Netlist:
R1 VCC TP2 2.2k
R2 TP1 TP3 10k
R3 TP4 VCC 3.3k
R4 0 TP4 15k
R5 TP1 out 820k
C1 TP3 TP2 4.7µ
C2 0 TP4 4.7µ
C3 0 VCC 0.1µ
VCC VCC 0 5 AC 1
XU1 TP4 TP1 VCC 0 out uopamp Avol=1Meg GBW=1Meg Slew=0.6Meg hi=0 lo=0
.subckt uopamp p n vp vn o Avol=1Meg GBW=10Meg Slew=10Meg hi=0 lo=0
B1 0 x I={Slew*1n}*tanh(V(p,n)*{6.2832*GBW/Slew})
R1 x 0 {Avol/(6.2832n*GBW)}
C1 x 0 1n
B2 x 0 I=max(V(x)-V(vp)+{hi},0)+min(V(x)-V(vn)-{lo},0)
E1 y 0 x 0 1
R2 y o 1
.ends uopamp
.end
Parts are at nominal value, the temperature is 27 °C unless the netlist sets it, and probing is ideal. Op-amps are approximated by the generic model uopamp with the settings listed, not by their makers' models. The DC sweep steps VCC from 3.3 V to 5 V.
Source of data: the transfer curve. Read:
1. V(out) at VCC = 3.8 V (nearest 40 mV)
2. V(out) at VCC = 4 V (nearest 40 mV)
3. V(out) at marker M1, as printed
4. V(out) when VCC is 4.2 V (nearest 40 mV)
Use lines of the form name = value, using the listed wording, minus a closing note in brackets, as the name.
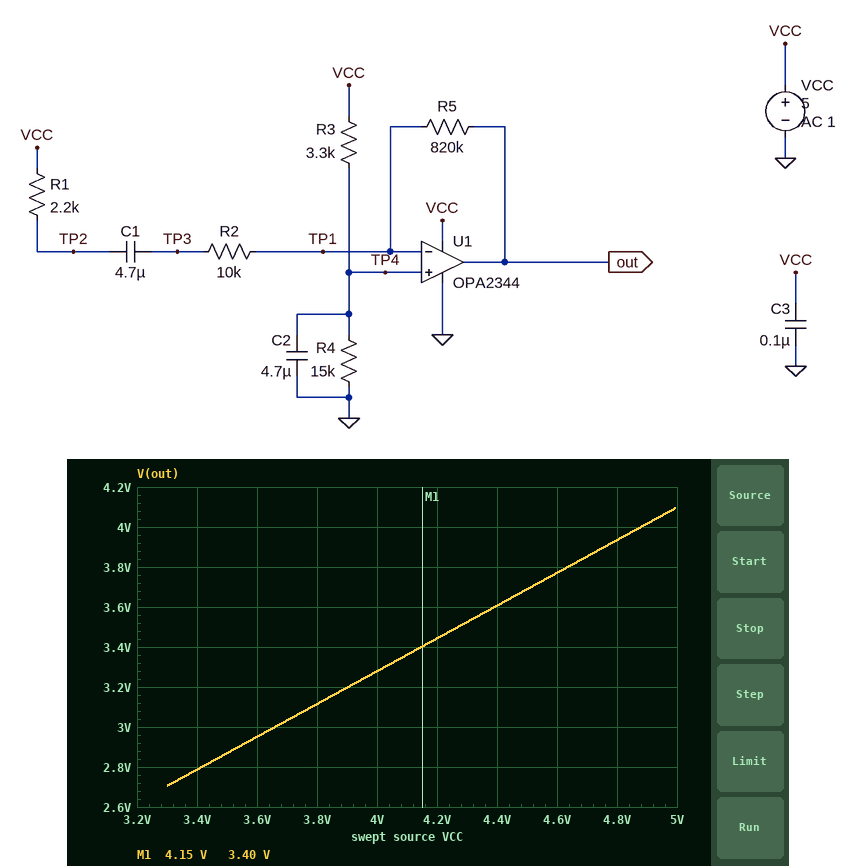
V(out) at VCC = 3.8 V = 3.12 V
V(out) at VCC = 4 V = 3.28 V
V(out) at marker M1, as printed = 3.40 V
V(out) when VCC is 4.2 V = 3.44 V
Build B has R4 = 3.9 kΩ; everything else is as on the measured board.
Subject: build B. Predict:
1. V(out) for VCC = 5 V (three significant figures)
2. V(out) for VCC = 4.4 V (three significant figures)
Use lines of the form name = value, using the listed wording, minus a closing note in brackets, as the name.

V(out) for VCC = 5 V = 2.71 V
V(out) for VCC = 4.4 V = 2.38 V
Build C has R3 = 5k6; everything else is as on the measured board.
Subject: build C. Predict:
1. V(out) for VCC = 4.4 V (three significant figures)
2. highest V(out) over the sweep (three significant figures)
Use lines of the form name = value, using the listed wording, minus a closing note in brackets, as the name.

V(out) for VCC = 4.4 V = 3.20 V
highest V(out) over the sweep = 3.64 V
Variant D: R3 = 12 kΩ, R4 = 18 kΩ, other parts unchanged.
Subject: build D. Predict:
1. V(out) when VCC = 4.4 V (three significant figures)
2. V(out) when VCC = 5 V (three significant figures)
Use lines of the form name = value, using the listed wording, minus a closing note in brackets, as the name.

V(out) when VCC = 4.4 V = 2.64 V
V(out) when VCC = 5 V = 3.00 V
